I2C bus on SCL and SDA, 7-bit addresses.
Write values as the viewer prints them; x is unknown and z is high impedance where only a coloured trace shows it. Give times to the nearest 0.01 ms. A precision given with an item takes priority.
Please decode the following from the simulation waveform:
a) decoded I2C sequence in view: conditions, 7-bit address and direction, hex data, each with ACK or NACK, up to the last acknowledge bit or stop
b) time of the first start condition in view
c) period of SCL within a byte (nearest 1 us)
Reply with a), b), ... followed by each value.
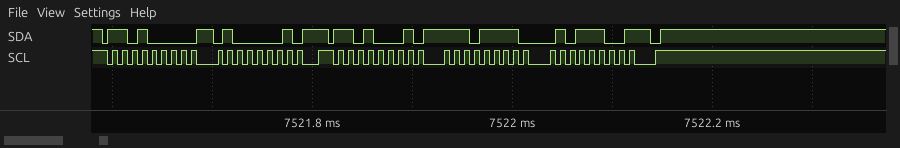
a) start, address 68 write ACK, 41 ACK, repeated start, address 68 read ACK, EF ACK, 5C NACK, stop
b) 7521.59 ms
c) 10 us
